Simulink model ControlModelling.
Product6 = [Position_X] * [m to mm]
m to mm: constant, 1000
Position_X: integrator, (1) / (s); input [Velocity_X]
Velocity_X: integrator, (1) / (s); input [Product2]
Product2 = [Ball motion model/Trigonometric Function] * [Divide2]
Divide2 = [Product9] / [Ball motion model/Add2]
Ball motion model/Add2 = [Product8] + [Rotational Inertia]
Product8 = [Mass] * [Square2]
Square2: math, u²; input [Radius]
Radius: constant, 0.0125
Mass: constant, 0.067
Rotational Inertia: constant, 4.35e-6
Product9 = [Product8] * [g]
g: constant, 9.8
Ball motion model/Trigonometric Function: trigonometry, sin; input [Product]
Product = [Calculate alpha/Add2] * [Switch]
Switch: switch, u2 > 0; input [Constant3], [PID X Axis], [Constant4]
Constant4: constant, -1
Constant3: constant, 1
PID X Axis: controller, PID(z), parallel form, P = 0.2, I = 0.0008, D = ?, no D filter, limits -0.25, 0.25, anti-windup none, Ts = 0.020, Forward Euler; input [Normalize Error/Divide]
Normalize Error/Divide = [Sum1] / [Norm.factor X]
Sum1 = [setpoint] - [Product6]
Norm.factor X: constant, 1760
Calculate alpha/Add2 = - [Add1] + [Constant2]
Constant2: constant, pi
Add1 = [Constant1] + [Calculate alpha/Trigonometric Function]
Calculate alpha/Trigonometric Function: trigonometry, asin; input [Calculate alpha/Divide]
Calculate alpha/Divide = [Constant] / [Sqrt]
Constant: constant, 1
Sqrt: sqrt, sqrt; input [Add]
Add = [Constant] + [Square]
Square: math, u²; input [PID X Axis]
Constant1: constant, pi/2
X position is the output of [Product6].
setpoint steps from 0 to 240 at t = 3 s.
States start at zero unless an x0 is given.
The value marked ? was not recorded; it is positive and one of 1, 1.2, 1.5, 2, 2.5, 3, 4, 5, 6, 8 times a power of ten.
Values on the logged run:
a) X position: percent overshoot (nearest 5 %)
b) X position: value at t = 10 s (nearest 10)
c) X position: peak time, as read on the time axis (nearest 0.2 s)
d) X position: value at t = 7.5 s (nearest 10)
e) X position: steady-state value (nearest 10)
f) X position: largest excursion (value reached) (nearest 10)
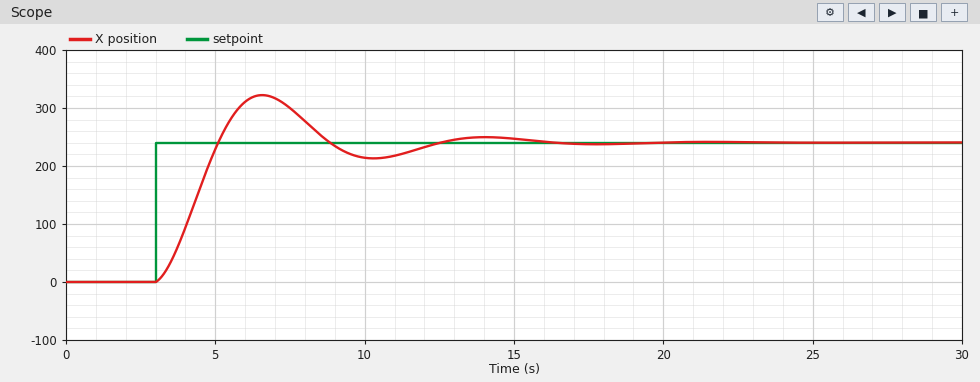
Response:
35 %
210
6.6 s
300
240
320
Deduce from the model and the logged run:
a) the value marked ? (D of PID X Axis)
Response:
0.15
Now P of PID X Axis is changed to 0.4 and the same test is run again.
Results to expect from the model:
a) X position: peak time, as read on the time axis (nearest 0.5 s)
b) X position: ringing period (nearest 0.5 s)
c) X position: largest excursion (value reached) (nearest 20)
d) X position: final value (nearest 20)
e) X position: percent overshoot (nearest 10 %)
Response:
5.5 s
5.0 s
360
240
50 %
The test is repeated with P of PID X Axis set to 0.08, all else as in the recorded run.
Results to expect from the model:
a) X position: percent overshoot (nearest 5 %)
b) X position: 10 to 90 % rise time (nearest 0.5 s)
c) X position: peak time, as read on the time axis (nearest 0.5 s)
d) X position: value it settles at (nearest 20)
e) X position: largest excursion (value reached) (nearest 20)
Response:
15 %
3.0 s
9.0 s
240
280
